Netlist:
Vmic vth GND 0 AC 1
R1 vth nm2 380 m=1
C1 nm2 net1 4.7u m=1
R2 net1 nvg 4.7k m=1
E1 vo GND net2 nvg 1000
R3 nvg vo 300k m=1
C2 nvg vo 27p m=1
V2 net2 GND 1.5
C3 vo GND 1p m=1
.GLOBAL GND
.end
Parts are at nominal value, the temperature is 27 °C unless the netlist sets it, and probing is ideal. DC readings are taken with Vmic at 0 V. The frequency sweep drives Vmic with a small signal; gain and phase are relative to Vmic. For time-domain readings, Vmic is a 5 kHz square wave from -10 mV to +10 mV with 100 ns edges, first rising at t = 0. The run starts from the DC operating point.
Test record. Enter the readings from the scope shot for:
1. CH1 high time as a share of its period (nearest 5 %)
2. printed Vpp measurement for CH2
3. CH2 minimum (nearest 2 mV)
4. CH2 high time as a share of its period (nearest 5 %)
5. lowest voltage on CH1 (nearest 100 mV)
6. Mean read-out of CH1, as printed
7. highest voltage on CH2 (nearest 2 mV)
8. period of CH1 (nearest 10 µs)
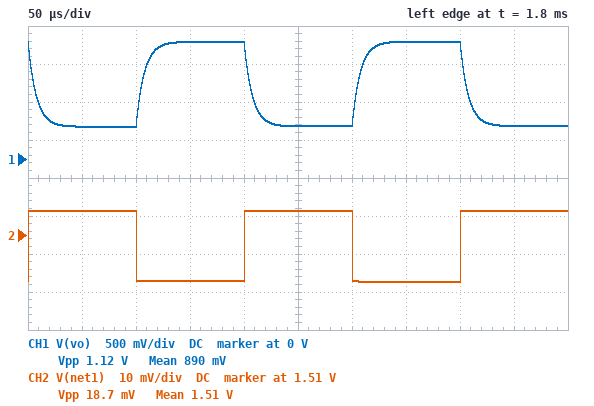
50 %
18.7 mV
1.498 V
50 %
400 mV
890 mV
1.516 V
200 µs
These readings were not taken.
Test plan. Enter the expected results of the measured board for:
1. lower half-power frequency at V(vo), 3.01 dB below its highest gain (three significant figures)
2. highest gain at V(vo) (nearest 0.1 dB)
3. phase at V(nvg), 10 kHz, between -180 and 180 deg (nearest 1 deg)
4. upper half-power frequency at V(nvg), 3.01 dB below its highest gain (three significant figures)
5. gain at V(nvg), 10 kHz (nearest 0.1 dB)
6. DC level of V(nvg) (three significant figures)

6.29 Hz
34.9 dB
-26 deg
20.8 kHz
-26.0 dB
1.50 V
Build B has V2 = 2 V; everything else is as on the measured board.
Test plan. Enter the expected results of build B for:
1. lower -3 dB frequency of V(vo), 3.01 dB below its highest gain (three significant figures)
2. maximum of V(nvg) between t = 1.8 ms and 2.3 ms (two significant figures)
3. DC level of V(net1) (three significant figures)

6.29 Hz
2.0 V
2.00 V
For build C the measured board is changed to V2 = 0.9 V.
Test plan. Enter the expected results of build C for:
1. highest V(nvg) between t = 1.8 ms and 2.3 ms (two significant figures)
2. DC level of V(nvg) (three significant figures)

900 mV
899 mV
